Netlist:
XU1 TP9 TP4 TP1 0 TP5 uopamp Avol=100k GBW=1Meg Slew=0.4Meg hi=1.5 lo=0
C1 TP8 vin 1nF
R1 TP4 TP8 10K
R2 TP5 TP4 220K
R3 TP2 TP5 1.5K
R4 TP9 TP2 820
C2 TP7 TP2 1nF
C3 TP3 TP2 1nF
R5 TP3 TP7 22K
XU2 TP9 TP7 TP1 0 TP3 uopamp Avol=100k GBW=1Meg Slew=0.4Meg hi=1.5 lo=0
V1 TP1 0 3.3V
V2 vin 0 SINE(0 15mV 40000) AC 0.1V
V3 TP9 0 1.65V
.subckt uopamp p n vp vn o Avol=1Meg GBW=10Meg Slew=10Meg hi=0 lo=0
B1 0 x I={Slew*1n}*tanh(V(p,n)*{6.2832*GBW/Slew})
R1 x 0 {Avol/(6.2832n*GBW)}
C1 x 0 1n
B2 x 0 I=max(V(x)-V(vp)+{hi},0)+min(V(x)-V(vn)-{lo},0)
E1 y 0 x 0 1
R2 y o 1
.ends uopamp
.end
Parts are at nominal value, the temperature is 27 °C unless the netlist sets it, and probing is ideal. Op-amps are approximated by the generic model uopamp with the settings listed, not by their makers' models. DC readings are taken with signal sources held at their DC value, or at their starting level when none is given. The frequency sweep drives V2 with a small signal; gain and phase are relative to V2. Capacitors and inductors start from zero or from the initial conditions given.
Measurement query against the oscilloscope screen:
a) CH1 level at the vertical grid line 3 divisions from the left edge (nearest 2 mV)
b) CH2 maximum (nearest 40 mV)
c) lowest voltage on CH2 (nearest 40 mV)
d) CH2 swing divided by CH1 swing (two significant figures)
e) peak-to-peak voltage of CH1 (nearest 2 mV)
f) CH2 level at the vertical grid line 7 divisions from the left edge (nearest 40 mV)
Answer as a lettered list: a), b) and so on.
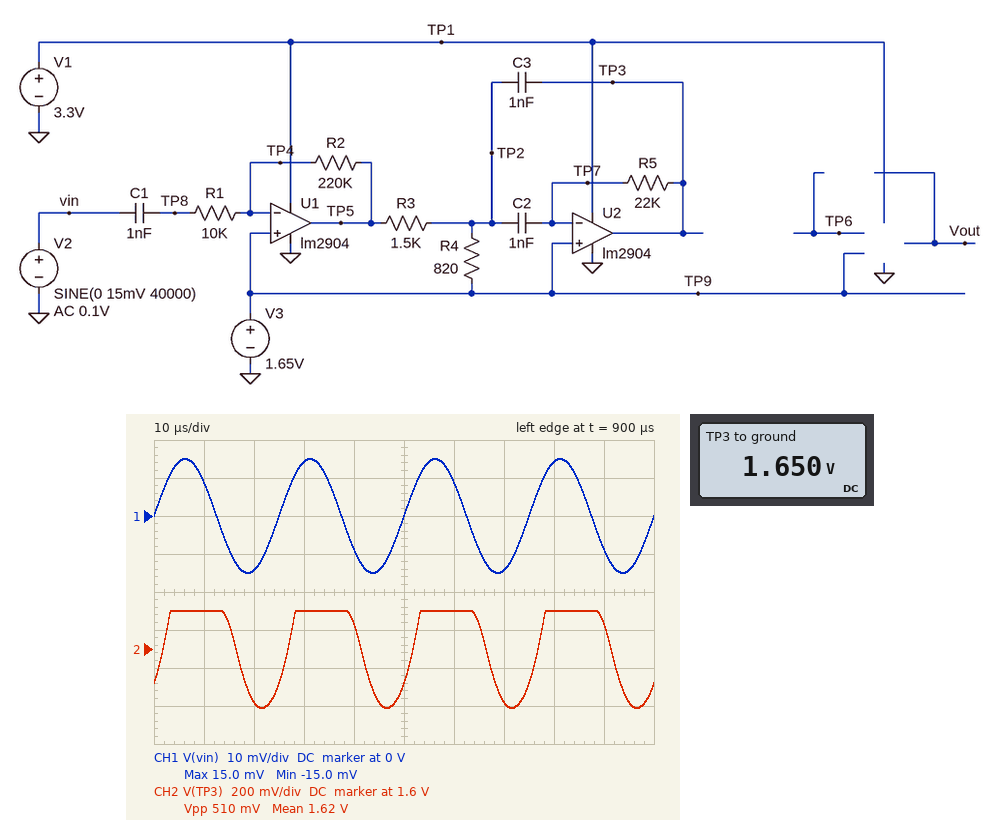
a) 14 mV
b) 1.80 V
c) 1.28 V
d) 17
e) 30 mV
f) 1.32 V
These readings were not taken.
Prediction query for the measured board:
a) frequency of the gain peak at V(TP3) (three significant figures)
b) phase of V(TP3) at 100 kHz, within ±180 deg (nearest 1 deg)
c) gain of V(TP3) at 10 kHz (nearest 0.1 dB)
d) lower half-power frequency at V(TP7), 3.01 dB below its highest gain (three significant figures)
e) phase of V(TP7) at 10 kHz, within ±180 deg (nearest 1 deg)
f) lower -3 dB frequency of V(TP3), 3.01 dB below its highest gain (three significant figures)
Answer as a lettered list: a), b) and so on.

a) 40.4 kHz
b) -151 deg
c) 16.5 dB
d) 36.1 kHz
e) 49 deg
f) 34.8 kHz
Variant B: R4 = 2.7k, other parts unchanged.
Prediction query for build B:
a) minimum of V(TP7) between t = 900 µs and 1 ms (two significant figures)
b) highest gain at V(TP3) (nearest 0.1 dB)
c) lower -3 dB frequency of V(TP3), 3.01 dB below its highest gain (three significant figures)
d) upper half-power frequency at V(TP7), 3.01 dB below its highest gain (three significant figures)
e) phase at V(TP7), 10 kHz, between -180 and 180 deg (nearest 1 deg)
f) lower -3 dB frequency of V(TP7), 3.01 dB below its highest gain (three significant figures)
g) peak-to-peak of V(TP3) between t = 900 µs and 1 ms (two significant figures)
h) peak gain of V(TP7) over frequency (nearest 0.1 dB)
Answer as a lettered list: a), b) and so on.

a) 1.5 V
b) 43.7 dB
c) 26.1 kHz
d) 40.9 kHz
e) 45 deg
f) 27.7 kHz
g) 520 mV
h) 13.9 dB
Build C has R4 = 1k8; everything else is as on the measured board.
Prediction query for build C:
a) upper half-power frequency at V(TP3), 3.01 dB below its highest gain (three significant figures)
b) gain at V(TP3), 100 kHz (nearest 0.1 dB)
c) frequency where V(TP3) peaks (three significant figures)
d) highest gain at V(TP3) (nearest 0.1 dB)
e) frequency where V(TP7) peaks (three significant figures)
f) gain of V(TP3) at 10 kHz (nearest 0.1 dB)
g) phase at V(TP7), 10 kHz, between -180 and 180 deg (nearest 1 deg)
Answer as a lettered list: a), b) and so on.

a) 40.0 kHz
b) 19.3 dB
c) 33.9 kHz
d) 43.5 dB
e) 35.0 kHz
f) 20.5 dB
g) 46 deg
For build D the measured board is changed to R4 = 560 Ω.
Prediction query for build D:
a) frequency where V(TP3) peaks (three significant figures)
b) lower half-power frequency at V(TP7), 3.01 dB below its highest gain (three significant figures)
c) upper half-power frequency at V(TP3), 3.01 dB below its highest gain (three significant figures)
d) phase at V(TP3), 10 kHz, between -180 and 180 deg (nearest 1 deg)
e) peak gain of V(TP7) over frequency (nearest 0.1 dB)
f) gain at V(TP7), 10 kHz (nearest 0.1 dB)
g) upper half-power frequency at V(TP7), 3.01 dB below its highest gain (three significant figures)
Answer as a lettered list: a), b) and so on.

a) 44.6 kHz
b) 40.3 kHz
c) 49.9 kHz
d) 140 deg
e) 15.0 dB
f) -25.8 dB
g) 51.3 kHz
